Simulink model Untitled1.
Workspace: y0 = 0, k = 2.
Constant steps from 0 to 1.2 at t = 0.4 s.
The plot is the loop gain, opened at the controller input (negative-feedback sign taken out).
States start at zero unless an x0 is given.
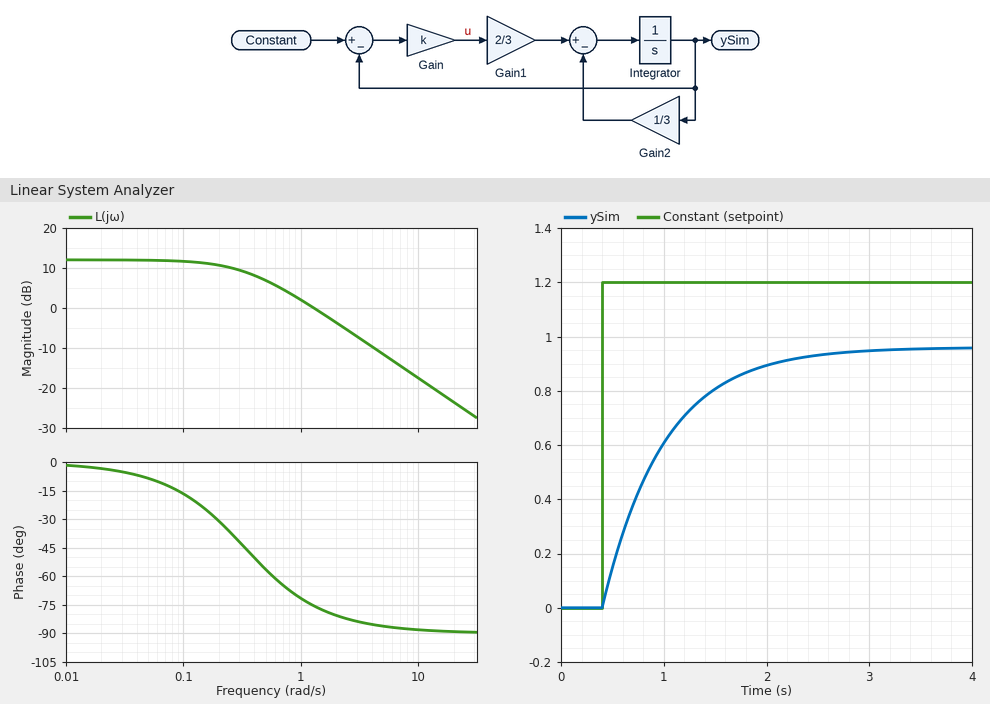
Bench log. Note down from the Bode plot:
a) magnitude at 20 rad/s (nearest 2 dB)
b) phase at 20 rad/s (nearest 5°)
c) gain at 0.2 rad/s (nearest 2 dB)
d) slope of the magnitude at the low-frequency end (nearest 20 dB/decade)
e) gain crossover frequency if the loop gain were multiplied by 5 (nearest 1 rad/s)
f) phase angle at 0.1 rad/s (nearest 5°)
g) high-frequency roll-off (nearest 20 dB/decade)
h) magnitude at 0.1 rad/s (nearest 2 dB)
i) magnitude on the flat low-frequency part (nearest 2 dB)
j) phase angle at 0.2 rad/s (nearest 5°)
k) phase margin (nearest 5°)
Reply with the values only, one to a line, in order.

-24 dB
-90°
10 dB
0 dB/decade
7 rad/s
-15°
-20 dB/decade
12 dB
12 dB
-30°
105°
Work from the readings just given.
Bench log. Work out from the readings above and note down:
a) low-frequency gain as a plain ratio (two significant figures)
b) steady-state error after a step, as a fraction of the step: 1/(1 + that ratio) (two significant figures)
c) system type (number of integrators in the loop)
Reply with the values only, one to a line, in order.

4.0
0.20
0
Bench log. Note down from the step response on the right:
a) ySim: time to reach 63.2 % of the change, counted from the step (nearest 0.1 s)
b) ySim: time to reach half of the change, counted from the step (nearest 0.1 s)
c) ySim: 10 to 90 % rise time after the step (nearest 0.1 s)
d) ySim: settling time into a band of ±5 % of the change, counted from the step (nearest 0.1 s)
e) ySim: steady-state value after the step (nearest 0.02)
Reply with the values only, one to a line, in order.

0.6 s
0.4 s
1.3 s
1.8 s
0.96
